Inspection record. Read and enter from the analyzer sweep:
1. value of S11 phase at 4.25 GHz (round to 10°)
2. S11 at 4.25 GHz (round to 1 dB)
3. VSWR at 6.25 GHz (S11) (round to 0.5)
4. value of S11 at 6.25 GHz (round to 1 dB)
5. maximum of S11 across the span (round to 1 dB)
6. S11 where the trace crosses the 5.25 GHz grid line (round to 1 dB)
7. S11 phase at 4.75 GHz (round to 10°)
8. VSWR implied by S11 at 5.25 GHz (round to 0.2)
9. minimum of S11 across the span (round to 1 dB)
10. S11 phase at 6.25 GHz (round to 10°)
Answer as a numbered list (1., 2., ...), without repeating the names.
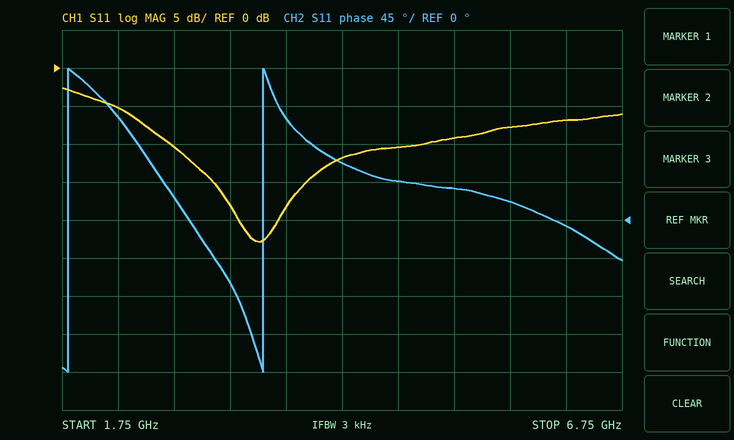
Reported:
1. 70°
2. -12 dB
3. 2.5
4. -7 dB
5. -3 dB
6. -9 dB
7. 50°
8. 2.0
9. -23 dB
10. -10°
